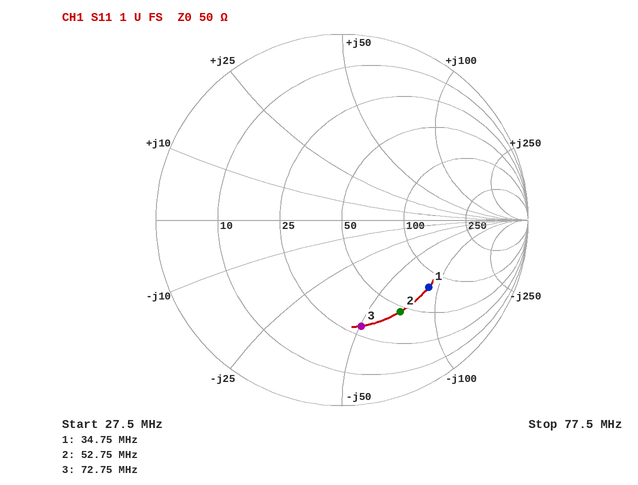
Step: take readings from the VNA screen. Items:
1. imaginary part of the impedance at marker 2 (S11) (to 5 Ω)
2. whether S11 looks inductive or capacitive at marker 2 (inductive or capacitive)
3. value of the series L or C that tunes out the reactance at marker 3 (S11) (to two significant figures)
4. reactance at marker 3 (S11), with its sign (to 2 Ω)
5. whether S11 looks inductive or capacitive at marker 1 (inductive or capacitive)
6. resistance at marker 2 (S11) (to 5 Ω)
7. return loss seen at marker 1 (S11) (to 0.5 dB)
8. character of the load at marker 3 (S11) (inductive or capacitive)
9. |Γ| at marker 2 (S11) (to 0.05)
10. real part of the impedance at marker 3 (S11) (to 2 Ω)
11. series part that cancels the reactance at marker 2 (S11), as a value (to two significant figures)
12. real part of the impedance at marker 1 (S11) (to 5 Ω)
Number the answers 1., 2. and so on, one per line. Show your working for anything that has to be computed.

1. -70 Ω
2. capacitive
3. L = 50 Ω/(2π × 72.75 MHz) ≈ 109 nH, so 110 nH to two significant figures
4. -50 Ω
5. capacitive
6. 45 Ω
7. 4.5 dB
8. capacitive
9. 0.60
10. 30 Ω
11. L = 70 Ω/(2π × 52.75 MHz) ≈ 211 nH, so 210 nH to two significant figures
12. 80 Ω
